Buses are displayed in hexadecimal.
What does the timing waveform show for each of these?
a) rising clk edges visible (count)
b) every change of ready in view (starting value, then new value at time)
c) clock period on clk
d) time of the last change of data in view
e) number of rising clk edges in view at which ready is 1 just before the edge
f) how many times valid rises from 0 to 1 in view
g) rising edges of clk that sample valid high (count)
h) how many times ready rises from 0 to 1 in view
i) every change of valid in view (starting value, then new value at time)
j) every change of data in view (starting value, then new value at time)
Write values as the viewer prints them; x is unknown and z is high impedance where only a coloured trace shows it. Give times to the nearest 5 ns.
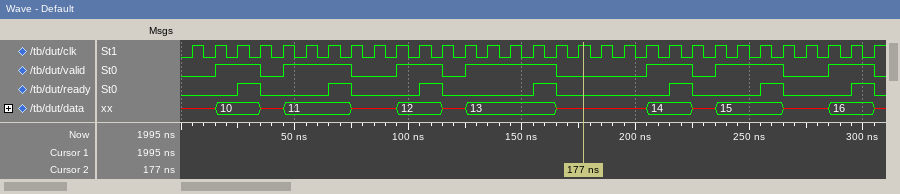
31
0, 1 at 25 ns, 0 at 35 ns, 1 at 65 ns, 0 at 75 ns, 1 at 105 ns, 0 at 115 ns, 1 at 155 ns, 0 at 165 ns, 1 at 215 ns, 0 at 225 ns, 1 at 255 ns, 0 at 265 ns, 1 at 295 ns, 0 at 305 ns
10 ns
305 ns
7
7
18
7
0, 1 at 15 ns, 0 at 35 ns, 1 at 45 ns, 0 at 75 ns, 1 at 95 ns, 0 at 115 ns, 1 at 125 ns, 0 at 165 ns, 1 at 205 ns, 0 at 225 ns, 1 at 235 ns, 0 at 265 ns, 1 at 285 ns, 0 at 305 ns
x, 10 at 15 ns, x at 35 ns, 11 at 45 ns, x at 75 ns, 12 at 95 ns, x at 115 ns, 13 at 125 ns, x at 165 ns, 14 at 205 ns, x at 225 ns, 15 at 235 ns, x at 265 ns, 16 at 285 ns, x at 305 ns
